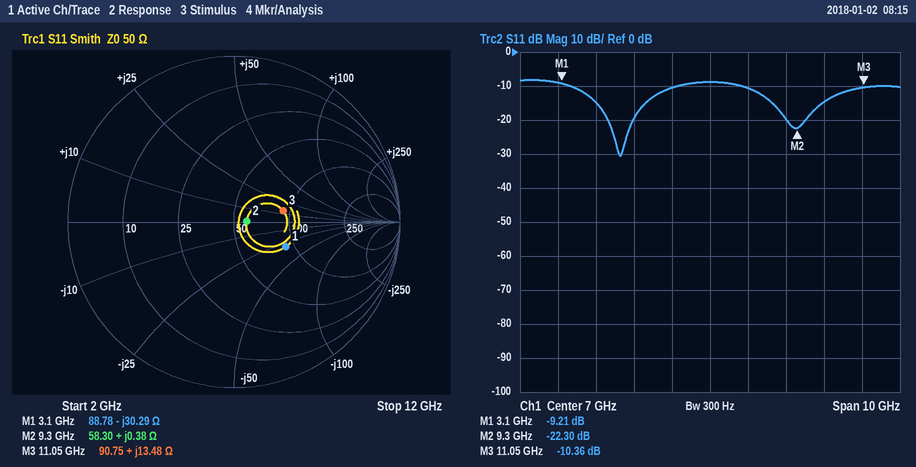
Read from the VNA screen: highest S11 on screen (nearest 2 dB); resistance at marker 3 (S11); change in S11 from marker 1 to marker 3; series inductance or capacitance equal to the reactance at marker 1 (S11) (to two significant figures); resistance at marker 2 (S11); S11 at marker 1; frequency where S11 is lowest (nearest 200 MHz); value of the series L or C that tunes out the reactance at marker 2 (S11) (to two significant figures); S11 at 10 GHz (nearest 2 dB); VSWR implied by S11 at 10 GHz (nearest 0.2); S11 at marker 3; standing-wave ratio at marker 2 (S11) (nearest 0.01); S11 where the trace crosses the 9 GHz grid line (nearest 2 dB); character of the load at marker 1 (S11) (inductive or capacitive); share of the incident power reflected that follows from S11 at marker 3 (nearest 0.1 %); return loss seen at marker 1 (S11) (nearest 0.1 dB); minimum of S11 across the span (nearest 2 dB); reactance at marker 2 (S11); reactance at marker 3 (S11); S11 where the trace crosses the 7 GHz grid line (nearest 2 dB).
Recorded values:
-8 dB
90.75 Ω
-1.15 dB
1.7 pF
58.30 Ω
-9.21 dB
4.6 GHz
45 pF
-14 dB
1.4
-10.36 dB
1.17
-20 dB
capacitive
9.2 %
9.2 dB
-30 dB
+0.38 Ω
+13.48 Ω
-8 dB
